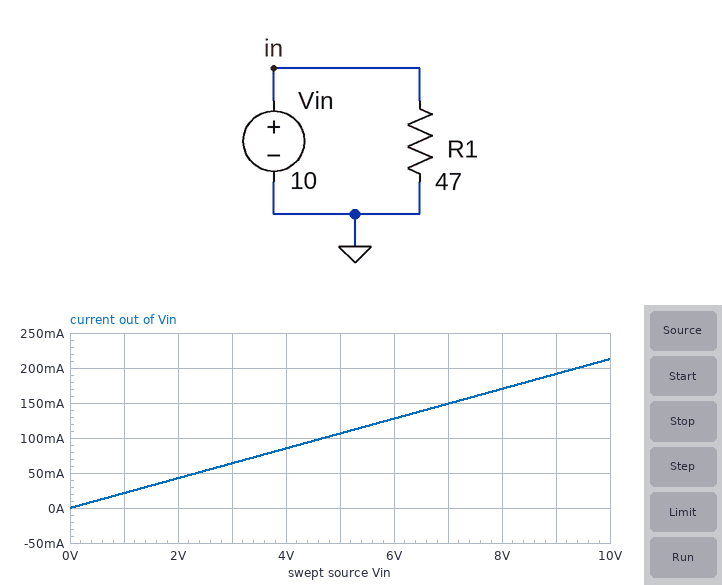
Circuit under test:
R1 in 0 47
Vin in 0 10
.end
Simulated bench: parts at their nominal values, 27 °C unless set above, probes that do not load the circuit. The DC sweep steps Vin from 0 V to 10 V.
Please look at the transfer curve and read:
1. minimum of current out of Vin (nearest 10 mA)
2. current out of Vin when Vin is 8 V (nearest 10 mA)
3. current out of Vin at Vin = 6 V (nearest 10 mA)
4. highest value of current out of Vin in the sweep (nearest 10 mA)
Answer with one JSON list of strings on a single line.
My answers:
["0 A", "170 mA", "130 mA", "210 mA"]
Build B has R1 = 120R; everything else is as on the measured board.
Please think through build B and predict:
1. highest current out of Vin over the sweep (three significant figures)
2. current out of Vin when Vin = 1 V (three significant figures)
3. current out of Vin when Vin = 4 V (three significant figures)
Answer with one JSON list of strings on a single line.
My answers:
["83.3 mA", "8.33 mA", "33.3 mA"]
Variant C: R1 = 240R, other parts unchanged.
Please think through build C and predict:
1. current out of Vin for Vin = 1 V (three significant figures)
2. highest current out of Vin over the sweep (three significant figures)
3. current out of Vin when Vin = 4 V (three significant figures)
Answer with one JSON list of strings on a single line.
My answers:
["4.17 mA", "41.7 mA", "16.7 mA"]
